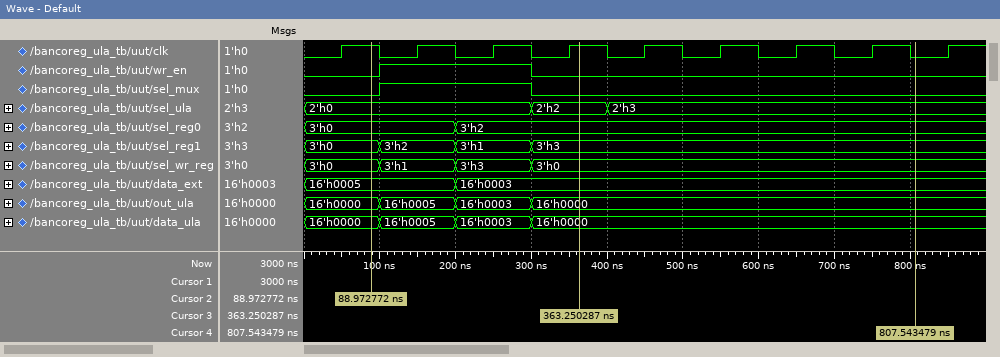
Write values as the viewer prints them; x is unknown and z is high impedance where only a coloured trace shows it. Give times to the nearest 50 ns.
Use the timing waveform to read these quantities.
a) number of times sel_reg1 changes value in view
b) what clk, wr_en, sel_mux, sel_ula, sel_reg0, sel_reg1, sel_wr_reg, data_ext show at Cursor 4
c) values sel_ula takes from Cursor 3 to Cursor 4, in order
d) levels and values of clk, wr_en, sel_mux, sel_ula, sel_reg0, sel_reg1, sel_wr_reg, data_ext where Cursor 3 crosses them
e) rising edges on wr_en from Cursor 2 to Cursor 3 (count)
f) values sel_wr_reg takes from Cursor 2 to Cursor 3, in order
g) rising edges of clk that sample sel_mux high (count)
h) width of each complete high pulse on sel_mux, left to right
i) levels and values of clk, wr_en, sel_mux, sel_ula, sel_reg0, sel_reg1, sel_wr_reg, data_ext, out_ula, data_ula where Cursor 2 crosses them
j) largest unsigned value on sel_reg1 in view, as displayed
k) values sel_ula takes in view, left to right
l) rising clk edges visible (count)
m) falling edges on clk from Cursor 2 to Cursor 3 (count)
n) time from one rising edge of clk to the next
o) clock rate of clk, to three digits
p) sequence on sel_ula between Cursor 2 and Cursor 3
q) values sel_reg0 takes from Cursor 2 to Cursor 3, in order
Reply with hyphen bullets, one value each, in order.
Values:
- 3
- clk=0, wr_en=0, sel_mux=0, sel_ula=2'h3, sel_reg0=3'h2, sel_reg1=3'h3, sel_wr_reg=3'h0, data_ext=16'h0003
- 2'h2, 2'h3
- clk=1, wr_en=0, sel_mux=0, sel_ula=2'h2, sel_reg0=3'h2, sel_reg1=3'h3, sel_wr_reg=3'h0, data_ext=16'h0003
- 1
- 3'h0, 3'h1, 3'h3, 3'h0
- 2
- 200 ns
- clk=1, wr_en=0, sel_mux=0, sel_ula=2'h0, sel_reg0=3'h0, sel_reg1=3'h0, sel_wr_reg=3'h0, data_ext=16'h0005, out_ula=16'h0000, data_ula=16'h0000
- 3'h3
- 2'h0, 2'h2, 2'h3
- 9
- 3
- 100 ns
- 10.0 MHz
- 2'h0, 2'h2
- 3'h0, 3'h2
